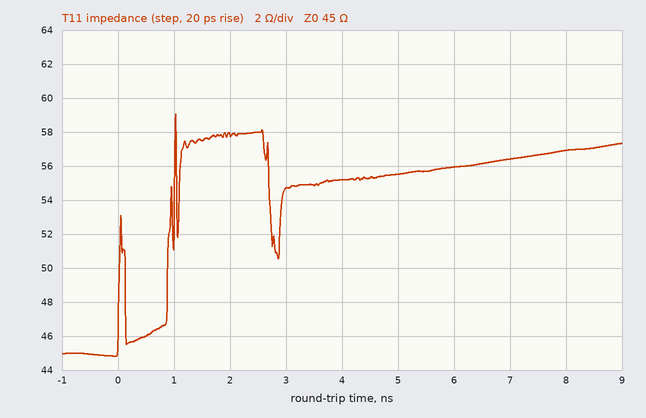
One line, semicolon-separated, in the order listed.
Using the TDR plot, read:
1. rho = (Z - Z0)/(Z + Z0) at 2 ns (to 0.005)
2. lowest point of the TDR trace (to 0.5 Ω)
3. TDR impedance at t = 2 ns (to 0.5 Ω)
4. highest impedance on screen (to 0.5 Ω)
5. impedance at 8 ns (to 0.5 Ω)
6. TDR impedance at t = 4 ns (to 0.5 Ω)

+0.125; 45.0 Ω; 58.0 Ω; 59.0 Ω; 57.0 Ω; 55.0 Ω
